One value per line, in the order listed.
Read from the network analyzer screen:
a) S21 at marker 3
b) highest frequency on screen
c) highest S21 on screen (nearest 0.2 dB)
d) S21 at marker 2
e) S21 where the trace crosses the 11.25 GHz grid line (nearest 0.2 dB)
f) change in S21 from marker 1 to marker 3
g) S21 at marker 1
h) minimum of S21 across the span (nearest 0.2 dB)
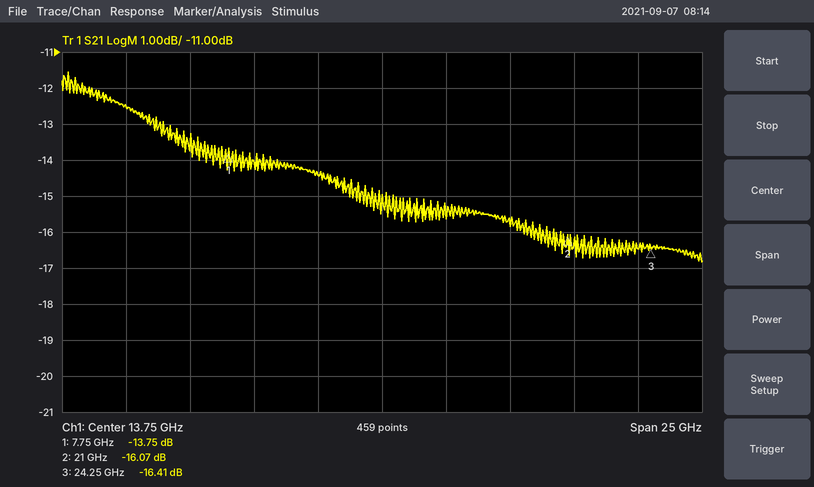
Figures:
-16.41 dB
26.25 GHz
-11.6 dB
-16.07 dB
-14.4 dB
-2.66 dB
-13.75 dB
-16.8 dB
